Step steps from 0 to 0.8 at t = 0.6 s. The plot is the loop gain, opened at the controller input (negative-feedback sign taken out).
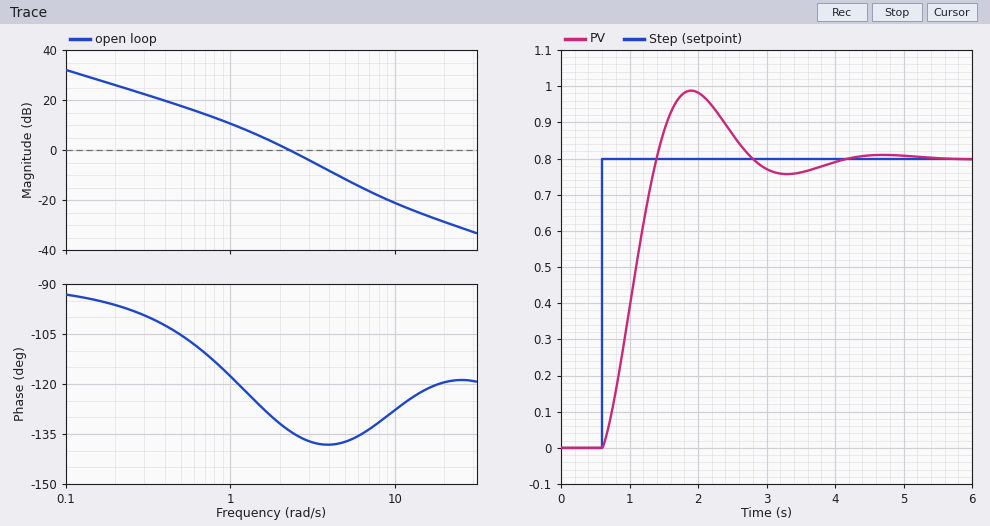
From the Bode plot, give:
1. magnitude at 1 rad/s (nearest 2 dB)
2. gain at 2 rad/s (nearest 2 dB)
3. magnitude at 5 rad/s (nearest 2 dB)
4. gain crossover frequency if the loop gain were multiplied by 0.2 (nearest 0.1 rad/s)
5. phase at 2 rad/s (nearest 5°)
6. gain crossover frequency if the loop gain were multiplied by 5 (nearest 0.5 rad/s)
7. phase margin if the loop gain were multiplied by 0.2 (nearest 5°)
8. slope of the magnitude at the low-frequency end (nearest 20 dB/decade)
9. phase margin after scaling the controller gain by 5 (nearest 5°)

10 dB
2 dB
-12 dB
0.7 rad/s
-130°
6.0 rad/s
70°
-20 dB/decade
45°
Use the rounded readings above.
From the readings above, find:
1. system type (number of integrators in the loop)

1
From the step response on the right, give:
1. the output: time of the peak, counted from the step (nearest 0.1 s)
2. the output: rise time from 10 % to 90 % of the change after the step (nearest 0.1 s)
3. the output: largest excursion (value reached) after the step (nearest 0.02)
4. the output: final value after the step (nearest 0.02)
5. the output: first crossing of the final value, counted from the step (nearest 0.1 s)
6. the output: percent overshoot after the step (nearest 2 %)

1.3 s
0.6 s
0.98
0.80
0.8 s
24 %
